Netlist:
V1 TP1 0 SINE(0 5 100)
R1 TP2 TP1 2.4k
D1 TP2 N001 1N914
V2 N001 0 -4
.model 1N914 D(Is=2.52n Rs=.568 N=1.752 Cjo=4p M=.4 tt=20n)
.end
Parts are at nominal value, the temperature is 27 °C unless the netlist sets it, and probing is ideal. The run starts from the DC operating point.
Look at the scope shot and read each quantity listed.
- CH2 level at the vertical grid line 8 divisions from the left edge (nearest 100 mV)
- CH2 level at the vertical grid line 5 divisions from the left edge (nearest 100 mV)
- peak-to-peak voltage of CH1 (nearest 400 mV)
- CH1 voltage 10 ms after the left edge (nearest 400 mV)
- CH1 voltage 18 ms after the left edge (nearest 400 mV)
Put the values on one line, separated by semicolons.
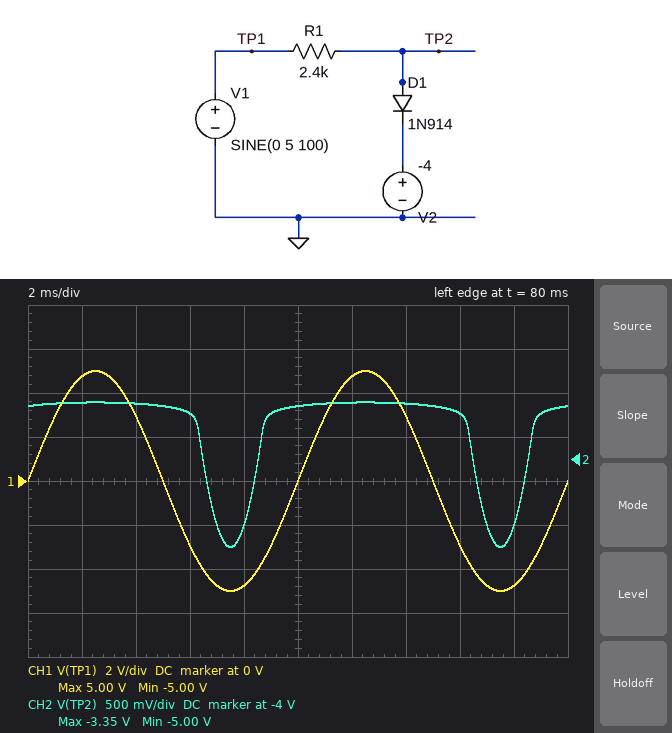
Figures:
-3.5 V; -3.4 V; 10.0 V; 0 V; -4.8 V
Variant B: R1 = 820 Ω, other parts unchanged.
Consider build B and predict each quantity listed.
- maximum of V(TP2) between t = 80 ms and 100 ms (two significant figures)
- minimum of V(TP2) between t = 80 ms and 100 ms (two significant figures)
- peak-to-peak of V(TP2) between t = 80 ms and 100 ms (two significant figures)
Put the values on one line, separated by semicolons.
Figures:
-3.3 V; -5.0 V; 1.7 V
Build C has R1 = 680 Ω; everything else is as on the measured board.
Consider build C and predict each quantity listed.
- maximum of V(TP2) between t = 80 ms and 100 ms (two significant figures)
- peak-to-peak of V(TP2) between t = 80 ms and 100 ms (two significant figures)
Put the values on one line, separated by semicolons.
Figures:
-3.3 V; 1.7 V
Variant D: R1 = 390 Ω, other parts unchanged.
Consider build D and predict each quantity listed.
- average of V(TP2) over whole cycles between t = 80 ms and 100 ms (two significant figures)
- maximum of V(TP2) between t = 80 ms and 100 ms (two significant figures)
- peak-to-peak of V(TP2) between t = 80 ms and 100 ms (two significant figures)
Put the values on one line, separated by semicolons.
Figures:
-3.6 V; -3.3 V; 1.7 V
